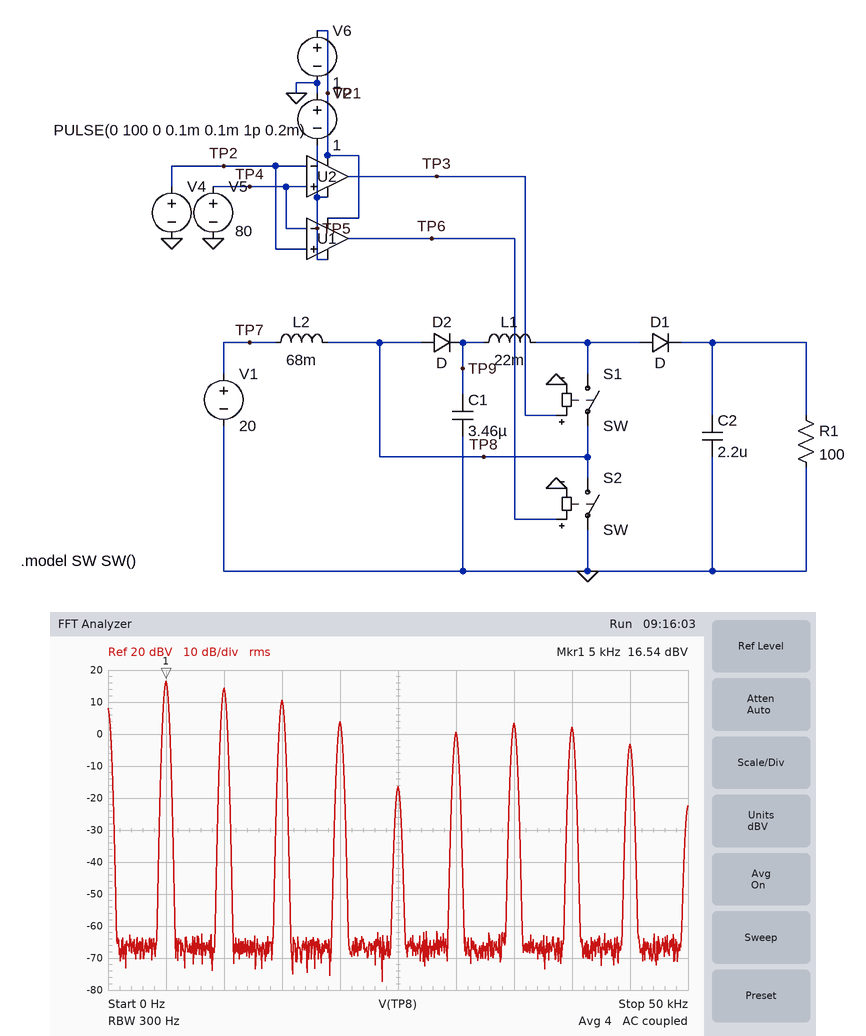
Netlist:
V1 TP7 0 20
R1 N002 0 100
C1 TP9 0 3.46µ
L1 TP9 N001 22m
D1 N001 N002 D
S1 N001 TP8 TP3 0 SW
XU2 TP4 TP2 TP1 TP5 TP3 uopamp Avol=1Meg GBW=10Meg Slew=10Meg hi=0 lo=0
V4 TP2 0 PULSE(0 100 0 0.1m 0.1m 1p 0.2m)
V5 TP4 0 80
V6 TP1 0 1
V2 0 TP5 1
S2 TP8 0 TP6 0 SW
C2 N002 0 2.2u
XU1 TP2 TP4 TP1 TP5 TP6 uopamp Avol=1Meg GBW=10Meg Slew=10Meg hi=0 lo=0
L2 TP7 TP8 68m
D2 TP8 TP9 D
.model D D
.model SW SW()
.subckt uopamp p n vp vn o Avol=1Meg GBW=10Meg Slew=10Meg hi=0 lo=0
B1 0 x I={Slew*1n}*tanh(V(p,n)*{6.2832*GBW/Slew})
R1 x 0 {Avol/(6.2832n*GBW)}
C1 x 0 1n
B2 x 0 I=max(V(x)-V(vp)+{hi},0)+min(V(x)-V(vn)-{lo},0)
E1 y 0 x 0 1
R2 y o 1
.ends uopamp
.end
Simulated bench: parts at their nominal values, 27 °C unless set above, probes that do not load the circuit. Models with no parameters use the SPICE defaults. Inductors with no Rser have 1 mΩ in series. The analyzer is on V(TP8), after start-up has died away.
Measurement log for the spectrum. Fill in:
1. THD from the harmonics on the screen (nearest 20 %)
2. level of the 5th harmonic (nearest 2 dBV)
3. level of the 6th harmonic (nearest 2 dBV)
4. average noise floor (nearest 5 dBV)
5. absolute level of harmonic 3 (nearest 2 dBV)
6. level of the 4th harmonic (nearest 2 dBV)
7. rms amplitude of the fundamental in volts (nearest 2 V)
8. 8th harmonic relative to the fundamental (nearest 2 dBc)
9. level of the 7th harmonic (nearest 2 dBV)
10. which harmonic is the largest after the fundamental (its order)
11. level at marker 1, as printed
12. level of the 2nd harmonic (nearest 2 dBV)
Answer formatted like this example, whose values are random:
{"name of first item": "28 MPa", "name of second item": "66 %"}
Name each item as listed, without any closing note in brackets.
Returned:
{"THD from the harmonics on the screen": "100 %", "level of the 5th harmonic": "-16 dBV", "level of the 6th harmonic": "0 dBV", "average noise floor": "-65 dBV", "absolute level of harmonic 3": "10 dBV", "level of the 4th harmonic": "4 dBV", "rms amplitude of the fundamental in volts": "6 V", "8th harmonic relative to the fundamental": "-14 dBc", "level of the 7th harmonic": "4 dBV", "which harmonic is the largest after the fundamental": "2", "level at marker 1, as printed": "16.54 dBV", "level of the 2nd harmonic": "14 dBV"}
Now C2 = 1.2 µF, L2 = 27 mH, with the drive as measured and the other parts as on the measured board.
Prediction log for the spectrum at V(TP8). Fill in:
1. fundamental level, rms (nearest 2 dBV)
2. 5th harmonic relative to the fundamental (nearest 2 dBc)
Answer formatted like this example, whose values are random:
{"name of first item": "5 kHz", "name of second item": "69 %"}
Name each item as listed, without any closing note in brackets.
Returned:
{"fundamental level, rms": "16 dBV", "5th harmonic relative to the fundamental": "-30 dBc"}
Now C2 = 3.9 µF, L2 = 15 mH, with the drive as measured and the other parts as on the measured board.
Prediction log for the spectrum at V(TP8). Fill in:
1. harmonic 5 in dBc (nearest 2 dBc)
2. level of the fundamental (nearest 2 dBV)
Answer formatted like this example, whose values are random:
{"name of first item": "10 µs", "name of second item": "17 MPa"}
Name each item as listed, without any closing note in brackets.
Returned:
{"harmonic 5 in dBc": "-36 dBc", "level of the fundamental": "16 dBV"}
